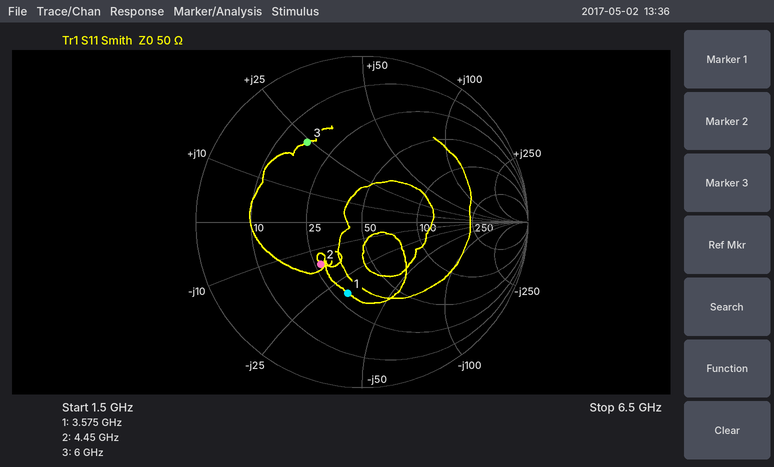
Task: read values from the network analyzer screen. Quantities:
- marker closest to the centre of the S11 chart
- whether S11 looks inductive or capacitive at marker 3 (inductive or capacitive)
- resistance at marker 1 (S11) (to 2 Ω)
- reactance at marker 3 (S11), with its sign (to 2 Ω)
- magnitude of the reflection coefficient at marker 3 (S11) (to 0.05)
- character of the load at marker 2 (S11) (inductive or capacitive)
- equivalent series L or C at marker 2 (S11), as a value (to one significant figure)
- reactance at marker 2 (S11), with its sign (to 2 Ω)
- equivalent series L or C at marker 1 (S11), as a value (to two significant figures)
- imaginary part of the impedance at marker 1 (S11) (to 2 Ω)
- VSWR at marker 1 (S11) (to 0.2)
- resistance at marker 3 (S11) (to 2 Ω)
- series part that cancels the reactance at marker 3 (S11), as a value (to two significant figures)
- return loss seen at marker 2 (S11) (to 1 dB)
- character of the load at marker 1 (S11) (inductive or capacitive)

marker 2
inductive
30 Ω
+24 Ω
0.60
capacitive
2 pF
-16 Ω
1.4 pF
-32 Ω
2.6
16 Ω
1.1 pF
9 dB
capacitive
